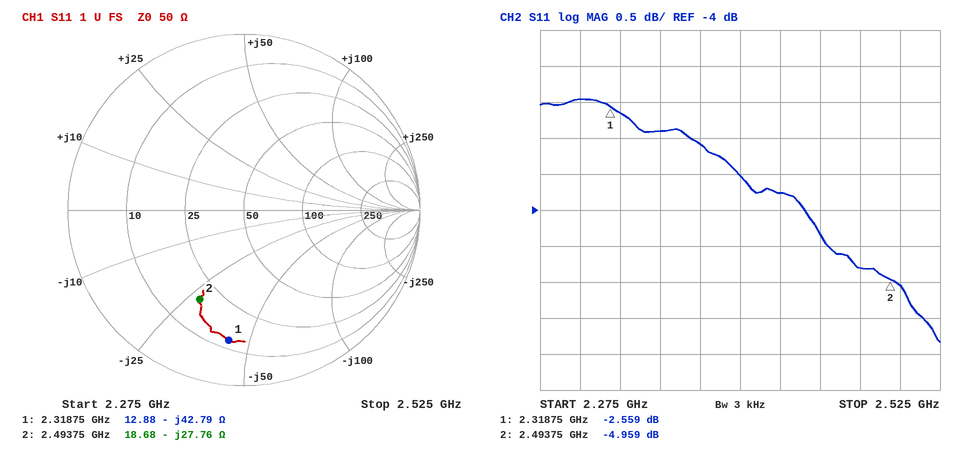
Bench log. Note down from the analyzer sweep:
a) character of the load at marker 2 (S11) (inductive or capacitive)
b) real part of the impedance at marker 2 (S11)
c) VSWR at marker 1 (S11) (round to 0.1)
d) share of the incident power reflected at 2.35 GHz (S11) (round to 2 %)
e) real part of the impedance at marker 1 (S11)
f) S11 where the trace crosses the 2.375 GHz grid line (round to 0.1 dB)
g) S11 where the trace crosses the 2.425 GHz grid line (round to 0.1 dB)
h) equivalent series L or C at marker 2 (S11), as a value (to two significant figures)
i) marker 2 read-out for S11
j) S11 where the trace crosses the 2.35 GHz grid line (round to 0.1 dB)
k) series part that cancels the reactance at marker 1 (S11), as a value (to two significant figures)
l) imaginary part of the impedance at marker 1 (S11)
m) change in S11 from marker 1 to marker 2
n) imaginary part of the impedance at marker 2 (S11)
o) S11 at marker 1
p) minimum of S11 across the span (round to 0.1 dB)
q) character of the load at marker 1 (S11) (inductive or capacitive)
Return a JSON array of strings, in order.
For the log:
["capacitive", "18.68 Ω", "6.8", "52 %", "12.88 Ω", "-3.1 dB", "-3.8 dB", "2.3 pF", "-4.959 dB", "-2.9 dB", "2.9 nH", "-42.79 Ω", "-2.400 dB", "-27.76 Ω", "-2.559 dB", "-5.8 dB", "capacitive"]
